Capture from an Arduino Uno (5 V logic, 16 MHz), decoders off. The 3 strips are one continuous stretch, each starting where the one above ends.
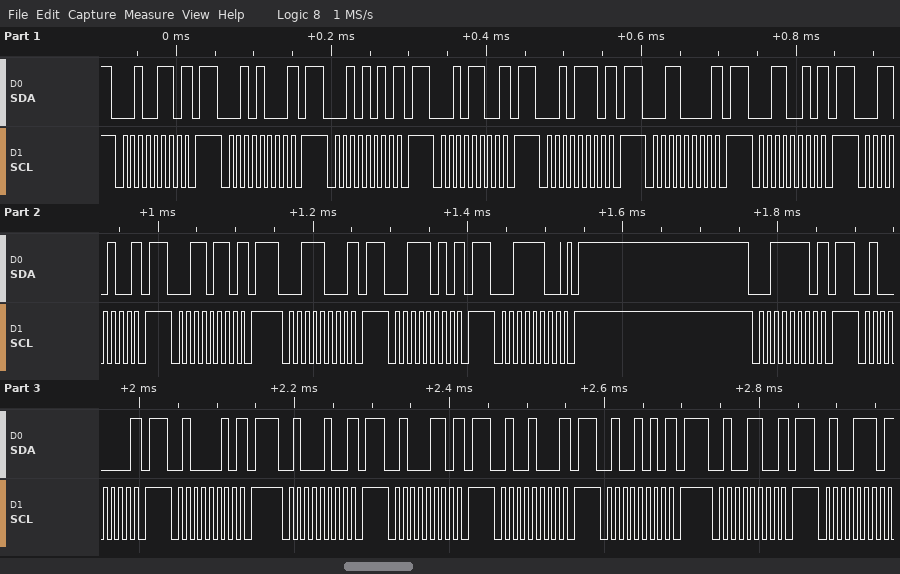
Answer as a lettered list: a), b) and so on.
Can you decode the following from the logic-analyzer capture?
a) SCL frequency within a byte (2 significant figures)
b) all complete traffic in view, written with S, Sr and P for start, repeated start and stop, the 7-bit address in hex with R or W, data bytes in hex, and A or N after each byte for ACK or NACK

a) 100 kHz
b) S 13W N P S 14W N P S 15W N P S 16W N P S 17W N P S 18W N P S 19W N P S 1AW N P S 1BW N P S 1CW N P S 1DW N P S 1EW A P S 1FW N P S 20W N P S 21W N P S 22W N P S 23W N P S 24W N P S 25W N P S 26W N P S 27W N
